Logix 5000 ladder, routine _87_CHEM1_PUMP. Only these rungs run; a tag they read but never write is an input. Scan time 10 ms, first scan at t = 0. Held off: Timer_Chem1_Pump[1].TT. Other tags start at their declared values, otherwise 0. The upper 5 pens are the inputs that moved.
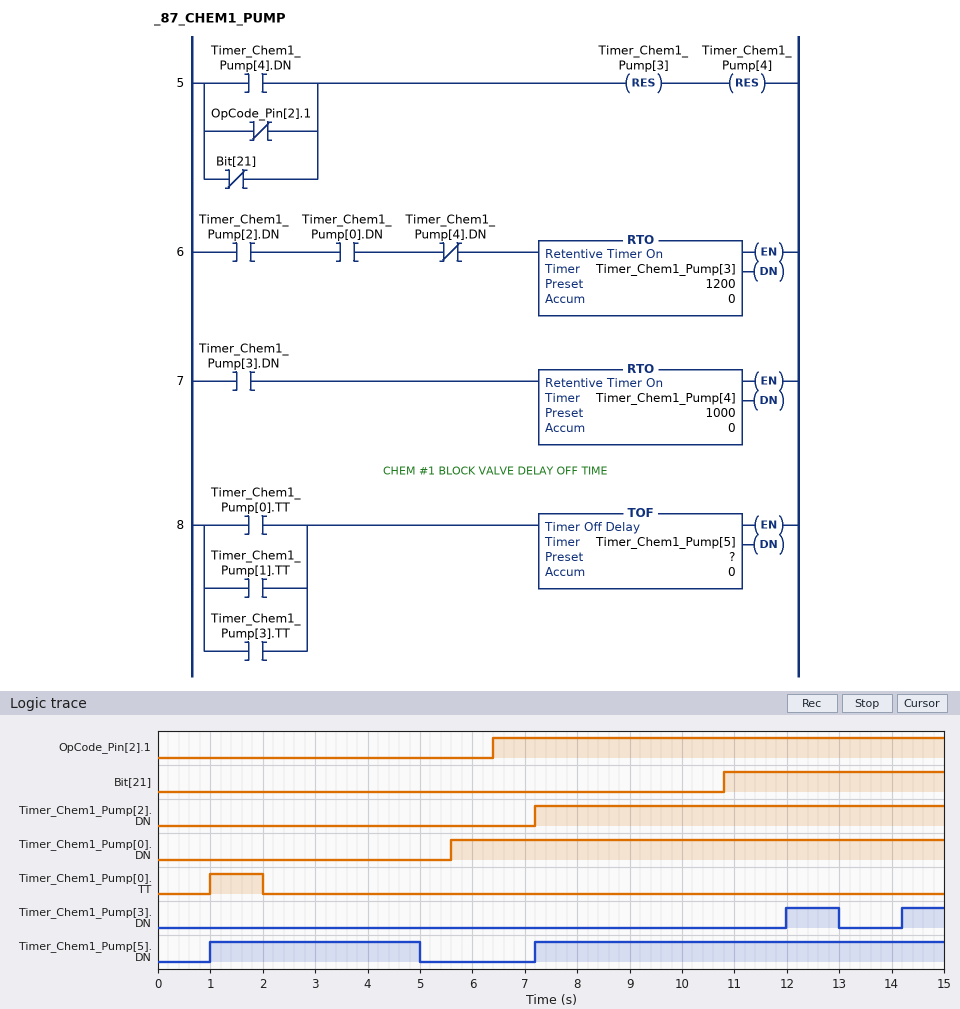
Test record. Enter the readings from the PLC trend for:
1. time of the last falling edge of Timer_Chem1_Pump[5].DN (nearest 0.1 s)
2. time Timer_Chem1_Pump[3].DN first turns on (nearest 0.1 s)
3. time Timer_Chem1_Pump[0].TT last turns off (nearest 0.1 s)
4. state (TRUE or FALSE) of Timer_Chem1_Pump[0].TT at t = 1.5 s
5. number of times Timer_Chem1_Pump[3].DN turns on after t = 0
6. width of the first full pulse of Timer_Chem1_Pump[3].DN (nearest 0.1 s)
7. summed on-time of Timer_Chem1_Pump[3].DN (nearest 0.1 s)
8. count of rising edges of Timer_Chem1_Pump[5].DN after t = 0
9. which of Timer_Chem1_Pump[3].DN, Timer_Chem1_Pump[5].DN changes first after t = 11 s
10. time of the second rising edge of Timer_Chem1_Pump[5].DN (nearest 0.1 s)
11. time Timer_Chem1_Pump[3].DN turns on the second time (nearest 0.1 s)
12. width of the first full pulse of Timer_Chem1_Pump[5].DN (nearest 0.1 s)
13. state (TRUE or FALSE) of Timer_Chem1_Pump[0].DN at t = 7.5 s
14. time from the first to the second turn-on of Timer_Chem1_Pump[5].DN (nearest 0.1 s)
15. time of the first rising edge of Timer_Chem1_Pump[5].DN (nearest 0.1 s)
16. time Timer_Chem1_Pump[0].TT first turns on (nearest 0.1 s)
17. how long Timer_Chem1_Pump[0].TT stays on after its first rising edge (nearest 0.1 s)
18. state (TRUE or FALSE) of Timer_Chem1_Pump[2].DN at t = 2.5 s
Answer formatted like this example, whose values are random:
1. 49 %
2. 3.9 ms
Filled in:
1. 5.0 s
2. 12.0 s
3. 2.0 s
4. TRUE
5. 2
6. 1.0 s
7. 1.8 s
8. 2
9. Timer_Chem1_Pump[3].DN
10. 7.2 s
11. 14.2 s
12. 4.0 s
13. TRUE
14. 6.2 s
15. 1.0 s
16. 1.0 s
17. 1.0 s
18. FALSE
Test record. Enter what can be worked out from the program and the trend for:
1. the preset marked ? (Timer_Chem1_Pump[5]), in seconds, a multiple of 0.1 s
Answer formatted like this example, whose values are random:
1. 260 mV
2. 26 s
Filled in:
1. 3.0 s
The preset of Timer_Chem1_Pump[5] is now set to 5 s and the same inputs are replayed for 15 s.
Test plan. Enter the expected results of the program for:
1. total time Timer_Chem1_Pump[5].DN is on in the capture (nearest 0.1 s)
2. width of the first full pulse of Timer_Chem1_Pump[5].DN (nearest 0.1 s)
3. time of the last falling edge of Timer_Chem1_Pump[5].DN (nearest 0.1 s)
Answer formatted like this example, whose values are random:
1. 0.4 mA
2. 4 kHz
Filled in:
1. 13.8 s
2. 6.0 s
3. 7.0 s
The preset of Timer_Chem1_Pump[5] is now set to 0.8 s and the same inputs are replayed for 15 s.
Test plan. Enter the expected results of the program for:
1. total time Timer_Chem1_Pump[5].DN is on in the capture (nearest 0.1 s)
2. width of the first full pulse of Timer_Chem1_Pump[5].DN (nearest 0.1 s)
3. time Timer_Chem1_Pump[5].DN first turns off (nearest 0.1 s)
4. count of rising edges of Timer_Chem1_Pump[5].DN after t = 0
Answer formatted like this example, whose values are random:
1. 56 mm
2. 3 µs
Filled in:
1. 9.4 s
2. 1.8 s
3. 2.8 s
4. 3
